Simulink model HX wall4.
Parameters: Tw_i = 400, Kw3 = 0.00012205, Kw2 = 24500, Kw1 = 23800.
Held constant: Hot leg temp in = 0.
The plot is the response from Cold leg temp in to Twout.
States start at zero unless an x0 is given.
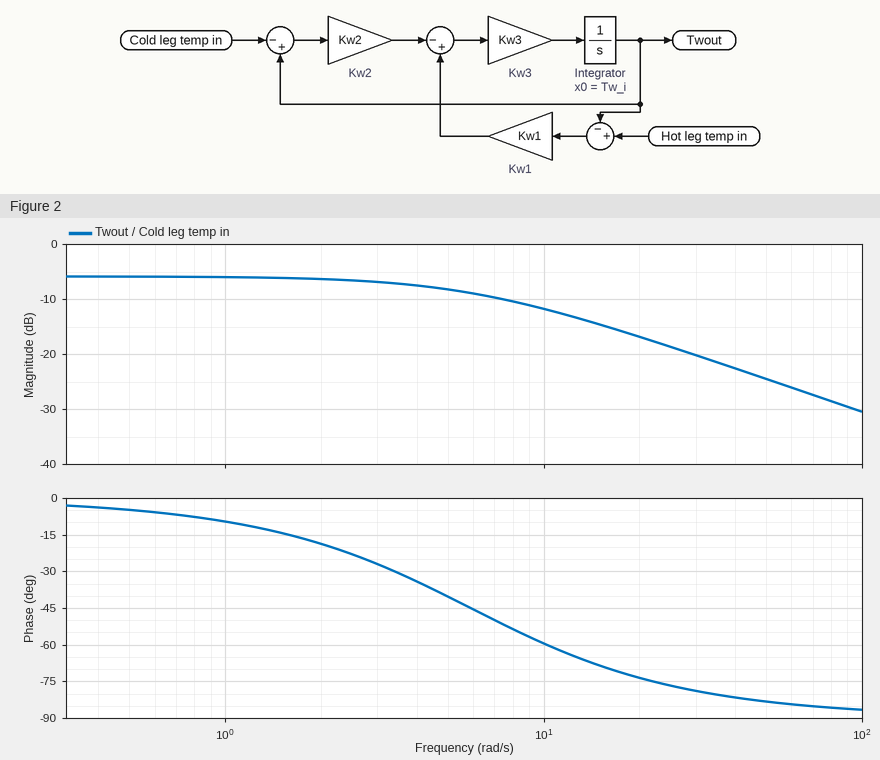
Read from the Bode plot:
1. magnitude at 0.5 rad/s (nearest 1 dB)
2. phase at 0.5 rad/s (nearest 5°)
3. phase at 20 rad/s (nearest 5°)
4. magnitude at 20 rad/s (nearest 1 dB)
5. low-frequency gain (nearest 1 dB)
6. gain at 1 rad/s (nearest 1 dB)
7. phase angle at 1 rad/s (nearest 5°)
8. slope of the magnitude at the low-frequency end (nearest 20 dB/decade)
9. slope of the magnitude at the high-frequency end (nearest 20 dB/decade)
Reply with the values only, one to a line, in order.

-6 dB
-5°
-75°
-17 dB
-6 dB
-6 dB
-10°
0 dB/decade
-20 dB/decade
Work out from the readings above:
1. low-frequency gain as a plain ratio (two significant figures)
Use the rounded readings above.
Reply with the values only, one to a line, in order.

0.50
